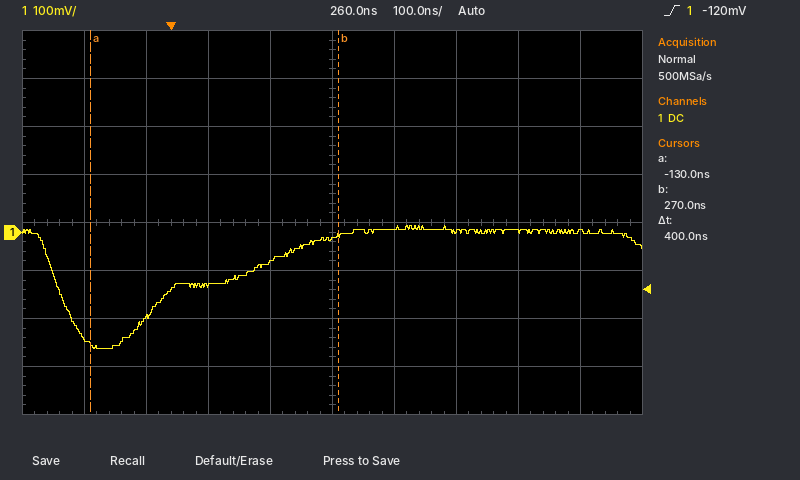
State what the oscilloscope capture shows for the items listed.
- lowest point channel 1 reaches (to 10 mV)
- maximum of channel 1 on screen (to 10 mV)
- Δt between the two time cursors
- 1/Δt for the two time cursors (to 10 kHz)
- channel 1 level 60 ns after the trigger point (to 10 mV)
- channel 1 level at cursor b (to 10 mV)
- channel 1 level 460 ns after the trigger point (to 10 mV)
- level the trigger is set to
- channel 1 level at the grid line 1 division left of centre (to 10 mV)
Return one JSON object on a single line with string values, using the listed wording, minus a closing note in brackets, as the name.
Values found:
{"lowest point channel 1 reaches": "-240 mV", "maximum of channel 1 on screen": "10 mV", "Δt between the two time cursors": "400 ns", "1/Δt for the two time cursors": "2.50 MHz", "channel 1 level 60 ns after the trigger point": "-110 mV", "channel 1 level at cursor b": "-10 mV", "channel 1 level 460 ns after the trigger point": "0 mV", "level the trigger is set to": "-120 mV", "channel 1 level at the grid line 1 division left of centre": "-60 mV"}
